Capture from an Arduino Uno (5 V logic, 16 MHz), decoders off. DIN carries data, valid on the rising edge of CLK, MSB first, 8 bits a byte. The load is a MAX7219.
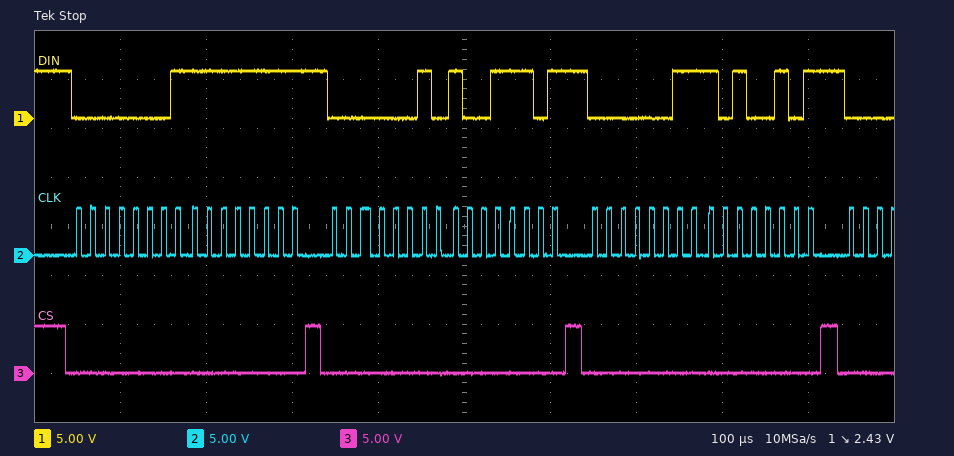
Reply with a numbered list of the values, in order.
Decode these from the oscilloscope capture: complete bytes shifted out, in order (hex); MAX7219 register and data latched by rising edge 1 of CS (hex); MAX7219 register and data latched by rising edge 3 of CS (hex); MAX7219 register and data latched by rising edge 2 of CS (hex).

1. 01 FF 02 9D 03 A5
2. register 0x1, data 0xFF
3. register 0x3, data 0xA5
4. register 0x2, data 0x9D
